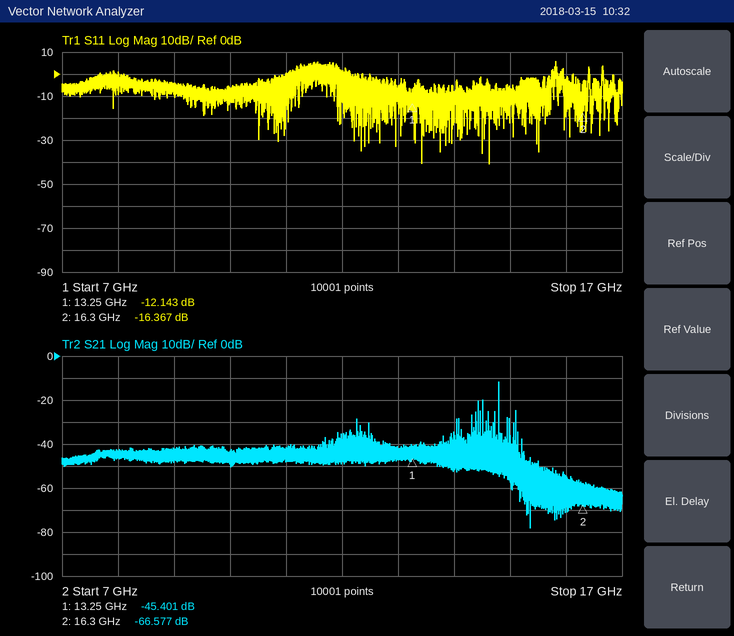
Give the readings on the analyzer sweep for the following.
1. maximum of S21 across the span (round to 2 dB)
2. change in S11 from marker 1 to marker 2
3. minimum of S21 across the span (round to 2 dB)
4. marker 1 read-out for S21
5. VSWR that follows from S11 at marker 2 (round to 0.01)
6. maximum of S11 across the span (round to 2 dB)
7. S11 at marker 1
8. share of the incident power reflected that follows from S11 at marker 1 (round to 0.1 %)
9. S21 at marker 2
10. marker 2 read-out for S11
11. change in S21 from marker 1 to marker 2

-12 dB
-4.224 dB
-78 dB
-45.401 dB
1.36
6 dB
-12.143 dB
6.1 %
-66.577 dB
-16.367 dB
-21.176 dB
